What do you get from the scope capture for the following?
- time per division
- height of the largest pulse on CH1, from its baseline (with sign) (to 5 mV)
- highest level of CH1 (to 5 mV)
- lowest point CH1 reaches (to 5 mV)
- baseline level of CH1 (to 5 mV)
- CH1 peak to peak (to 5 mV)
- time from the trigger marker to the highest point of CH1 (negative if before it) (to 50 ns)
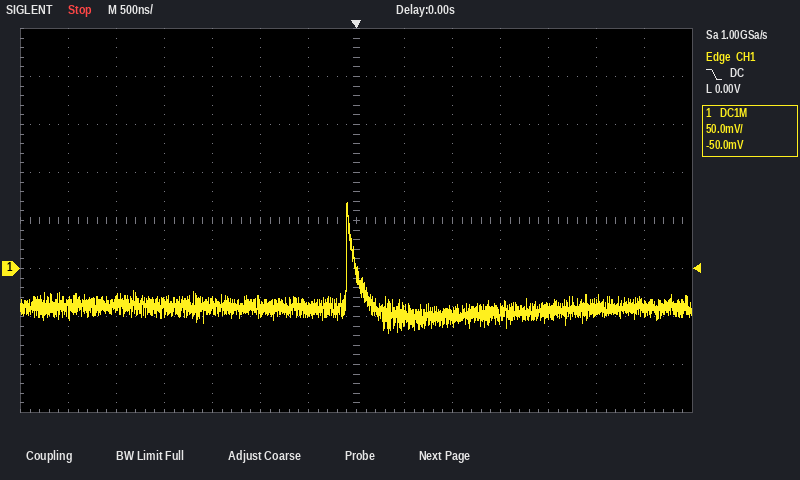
500 ns
+110 mV
70 mV
-65 mV
-40 mV
135 mV
-100 ns
